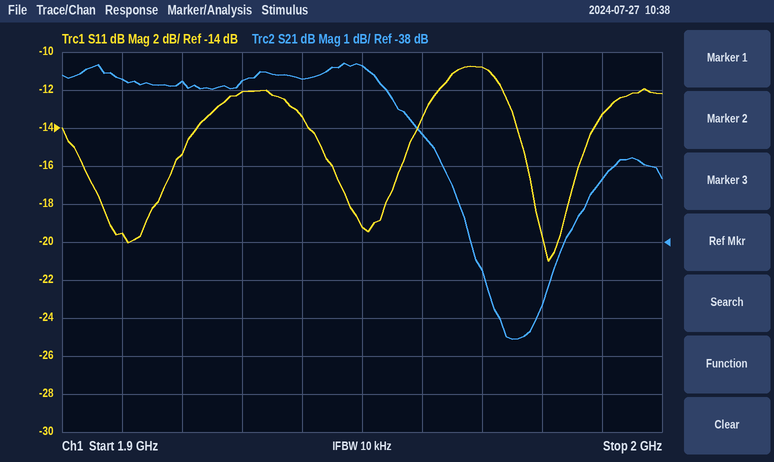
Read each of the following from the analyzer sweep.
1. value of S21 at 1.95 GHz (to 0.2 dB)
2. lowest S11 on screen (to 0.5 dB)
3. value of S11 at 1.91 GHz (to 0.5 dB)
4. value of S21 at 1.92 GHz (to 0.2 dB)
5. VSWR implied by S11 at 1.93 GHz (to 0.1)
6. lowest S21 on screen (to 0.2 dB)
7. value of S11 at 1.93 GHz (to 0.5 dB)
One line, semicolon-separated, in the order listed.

-33.4 dB; -21.0 dB; -19.5 dB; -33.8 dB; 1.7; -40.6 dB; -12.0 dB
